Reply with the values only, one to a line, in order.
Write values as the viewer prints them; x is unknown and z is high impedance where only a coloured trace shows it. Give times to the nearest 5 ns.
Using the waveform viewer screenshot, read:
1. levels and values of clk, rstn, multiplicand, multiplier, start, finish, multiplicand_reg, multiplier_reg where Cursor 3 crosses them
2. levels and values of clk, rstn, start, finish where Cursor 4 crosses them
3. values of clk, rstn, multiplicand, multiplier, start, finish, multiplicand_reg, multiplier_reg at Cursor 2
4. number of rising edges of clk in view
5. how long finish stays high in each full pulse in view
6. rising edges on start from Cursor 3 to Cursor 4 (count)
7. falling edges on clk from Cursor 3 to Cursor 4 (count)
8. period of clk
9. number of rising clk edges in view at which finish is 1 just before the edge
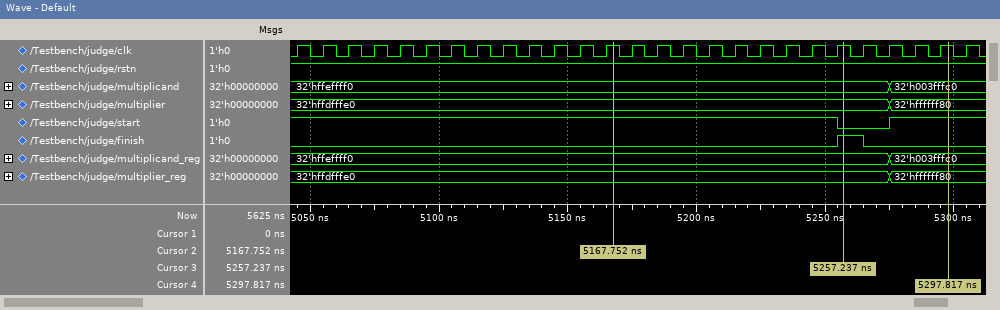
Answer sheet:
clk=1, rstn=1, multiplicand=32'hffeffff0, multiplier=32'hffdfffe0, start=0, finish=1, multiplicand_reg=32'hffeffff0, multiplier_reg=32'hffdfffe0
clk=1, rstn=1, start=1, finish=0
clk=1, rstn=1, multiplicand=32'hffeffff0, multiplier=32'hffdfffe0, start=1, finish=0, multiplicand_reg=32'hffeffff0, multiplier_reg=32'hffdfffe0
27
10 ns
1
4
10 ns
1
